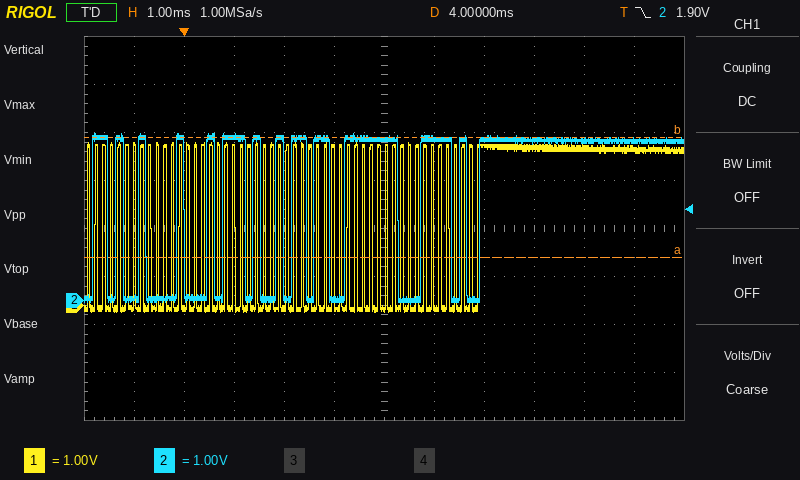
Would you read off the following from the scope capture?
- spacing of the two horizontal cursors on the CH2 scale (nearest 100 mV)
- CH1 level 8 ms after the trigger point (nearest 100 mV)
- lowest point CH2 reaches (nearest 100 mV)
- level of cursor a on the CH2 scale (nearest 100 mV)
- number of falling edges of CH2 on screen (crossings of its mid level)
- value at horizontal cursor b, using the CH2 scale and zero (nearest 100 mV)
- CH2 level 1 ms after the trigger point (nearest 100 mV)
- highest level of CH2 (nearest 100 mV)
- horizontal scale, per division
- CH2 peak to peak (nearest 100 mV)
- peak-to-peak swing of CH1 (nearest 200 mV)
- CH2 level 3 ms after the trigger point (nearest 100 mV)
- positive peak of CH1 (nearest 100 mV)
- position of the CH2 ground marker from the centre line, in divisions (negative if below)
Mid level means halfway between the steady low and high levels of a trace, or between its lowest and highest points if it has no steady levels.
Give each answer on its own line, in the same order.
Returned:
2.5 V
3.3 V
-100 mV
900 mV
13
3.4 V
3.4 V
3.5 V
1 ms
3.6 V
3.6 V
0.0 V
3.4 V
-1.5 div
